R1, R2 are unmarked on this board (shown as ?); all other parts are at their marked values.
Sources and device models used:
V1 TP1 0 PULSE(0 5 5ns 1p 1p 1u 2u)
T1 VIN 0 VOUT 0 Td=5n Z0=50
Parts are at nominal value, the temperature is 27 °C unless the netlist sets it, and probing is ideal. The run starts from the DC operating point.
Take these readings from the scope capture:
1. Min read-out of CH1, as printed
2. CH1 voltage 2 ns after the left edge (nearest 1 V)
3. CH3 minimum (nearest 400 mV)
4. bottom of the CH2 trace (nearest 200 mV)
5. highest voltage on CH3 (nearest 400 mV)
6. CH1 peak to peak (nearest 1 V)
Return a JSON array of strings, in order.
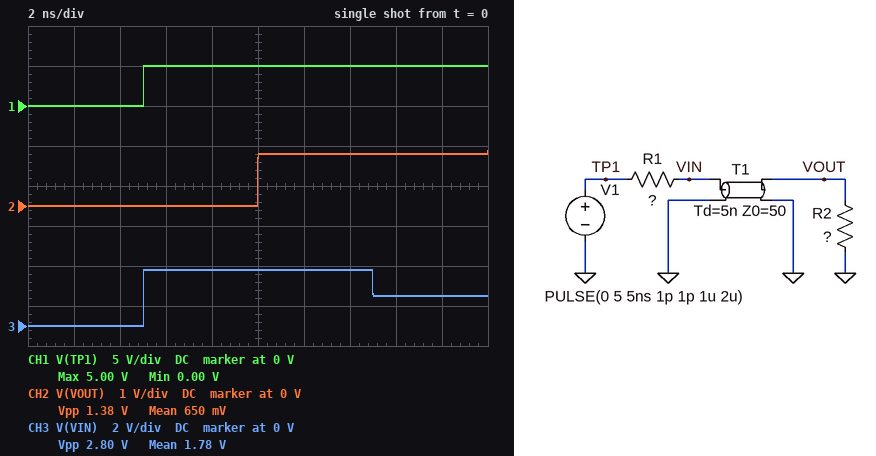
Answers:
["0.00 V", "0 V", "0 V", "0 V", "2.8 V", "5 V"]
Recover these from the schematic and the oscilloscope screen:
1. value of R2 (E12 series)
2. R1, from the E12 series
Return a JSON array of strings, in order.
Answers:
["15 Ω", "39 Ω"]
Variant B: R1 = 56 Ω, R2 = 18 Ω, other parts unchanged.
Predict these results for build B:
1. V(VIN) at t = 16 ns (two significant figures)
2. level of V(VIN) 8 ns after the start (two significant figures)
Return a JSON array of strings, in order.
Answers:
["1.2 V", "2.4 V"]
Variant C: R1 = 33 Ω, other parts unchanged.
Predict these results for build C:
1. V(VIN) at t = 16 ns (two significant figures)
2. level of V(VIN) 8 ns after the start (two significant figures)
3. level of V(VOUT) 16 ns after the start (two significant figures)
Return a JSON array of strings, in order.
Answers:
["1.7 V", "3.0 V", "1.4 V"]
